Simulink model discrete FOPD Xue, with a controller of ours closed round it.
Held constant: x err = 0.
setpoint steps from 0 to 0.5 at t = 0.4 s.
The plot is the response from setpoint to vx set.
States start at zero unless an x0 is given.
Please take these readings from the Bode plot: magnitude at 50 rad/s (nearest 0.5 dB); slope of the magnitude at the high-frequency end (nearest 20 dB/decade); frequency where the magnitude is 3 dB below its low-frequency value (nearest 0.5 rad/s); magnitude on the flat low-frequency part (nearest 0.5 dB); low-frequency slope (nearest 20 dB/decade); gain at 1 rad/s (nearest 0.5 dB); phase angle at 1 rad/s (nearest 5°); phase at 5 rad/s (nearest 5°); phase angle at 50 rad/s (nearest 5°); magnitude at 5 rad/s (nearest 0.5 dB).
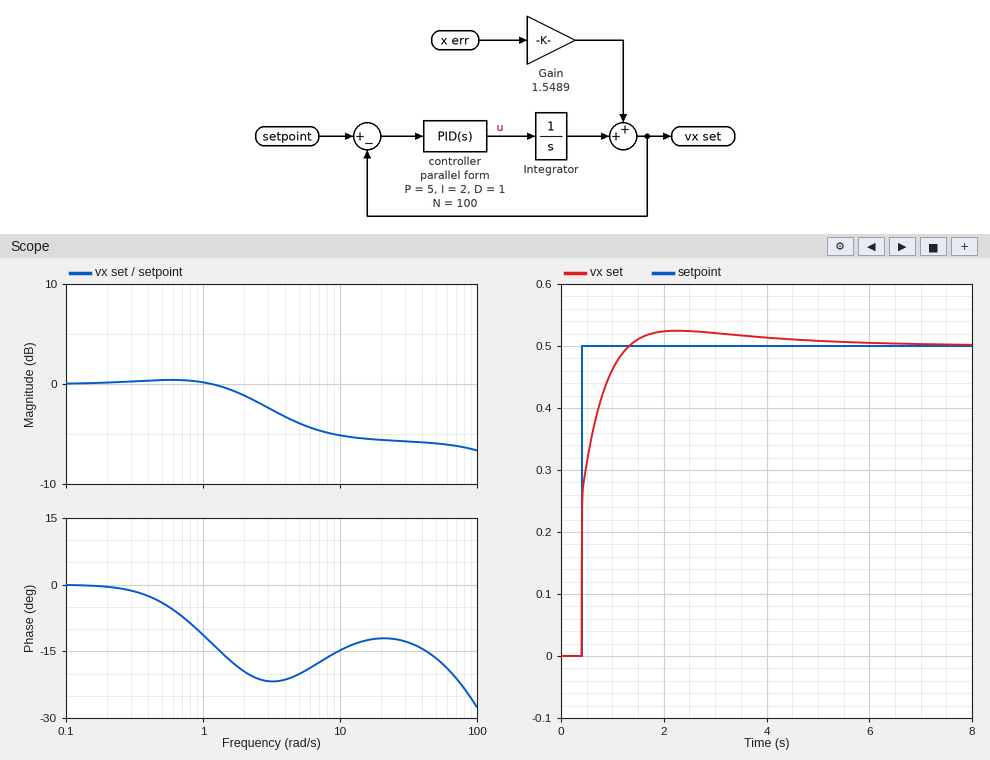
-6.0 dB
0 dB/decade
3.5 rad/s
0.0 dB
0 dB/decade
0.0 dB
-10°
-20°
-15°
-4.0 dB
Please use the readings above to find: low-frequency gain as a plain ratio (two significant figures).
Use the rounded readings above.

1.0
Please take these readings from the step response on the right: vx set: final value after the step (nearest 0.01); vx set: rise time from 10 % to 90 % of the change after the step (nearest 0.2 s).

0.50
0.6 s
